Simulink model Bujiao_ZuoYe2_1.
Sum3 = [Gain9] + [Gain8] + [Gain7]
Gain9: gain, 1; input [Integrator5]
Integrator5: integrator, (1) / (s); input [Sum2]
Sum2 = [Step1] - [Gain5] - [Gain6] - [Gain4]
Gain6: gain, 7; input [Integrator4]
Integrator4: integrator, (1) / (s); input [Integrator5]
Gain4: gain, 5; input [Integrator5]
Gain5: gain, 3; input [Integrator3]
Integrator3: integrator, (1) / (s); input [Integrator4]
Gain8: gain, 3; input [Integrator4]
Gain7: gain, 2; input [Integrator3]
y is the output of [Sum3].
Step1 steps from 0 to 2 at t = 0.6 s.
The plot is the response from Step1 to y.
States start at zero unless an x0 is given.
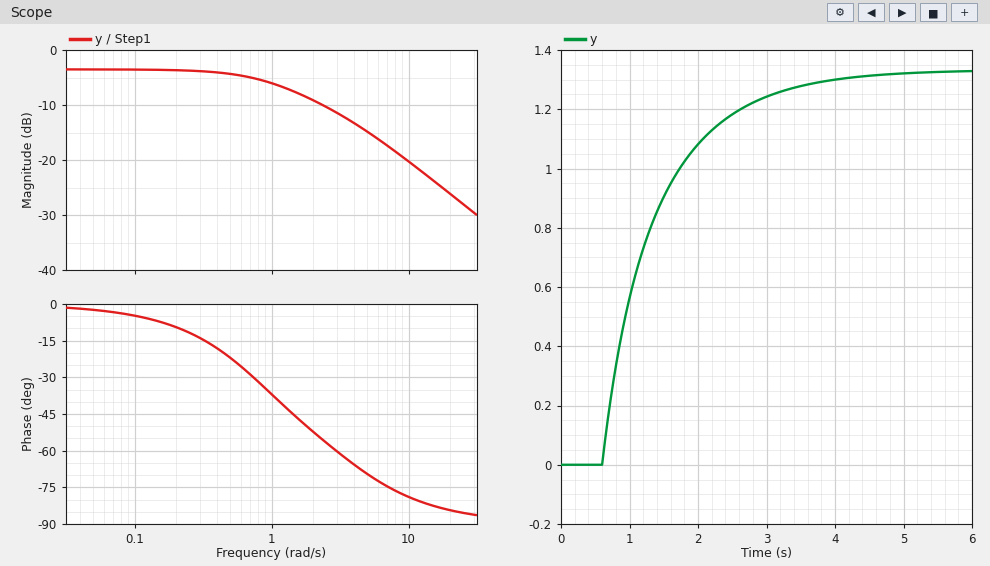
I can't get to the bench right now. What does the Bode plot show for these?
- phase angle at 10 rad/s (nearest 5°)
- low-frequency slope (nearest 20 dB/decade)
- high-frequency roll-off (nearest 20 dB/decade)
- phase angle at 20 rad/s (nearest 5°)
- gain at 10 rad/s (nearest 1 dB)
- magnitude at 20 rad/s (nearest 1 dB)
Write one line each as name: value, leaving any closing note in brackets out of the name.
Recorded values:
phase angle at 10 rad/s: -80°
low-frequency slope: 0 dB/decade
high-frequency roll-off: -20 dB/decade
phase angle at 20 rad/s: -85°
gain at 10 rad/s: -20 dB
magnitude at 20 rad/s: -26 dB
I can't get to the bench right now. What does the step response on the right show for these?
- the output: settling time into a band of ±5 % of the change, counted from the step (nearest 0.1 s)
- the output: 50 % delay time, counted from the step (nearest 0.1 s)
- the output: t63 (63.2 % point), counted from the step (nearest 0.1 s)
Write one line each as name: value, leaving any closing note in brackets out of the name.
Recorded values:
the output: settling time into a band of ±5 % of the change, counted from the step: 2.7 s
the output: 50 % delay time, counted from the step: 0.5 s
the output: t63 (63.2 % point), counted from the step: 0.8 s
